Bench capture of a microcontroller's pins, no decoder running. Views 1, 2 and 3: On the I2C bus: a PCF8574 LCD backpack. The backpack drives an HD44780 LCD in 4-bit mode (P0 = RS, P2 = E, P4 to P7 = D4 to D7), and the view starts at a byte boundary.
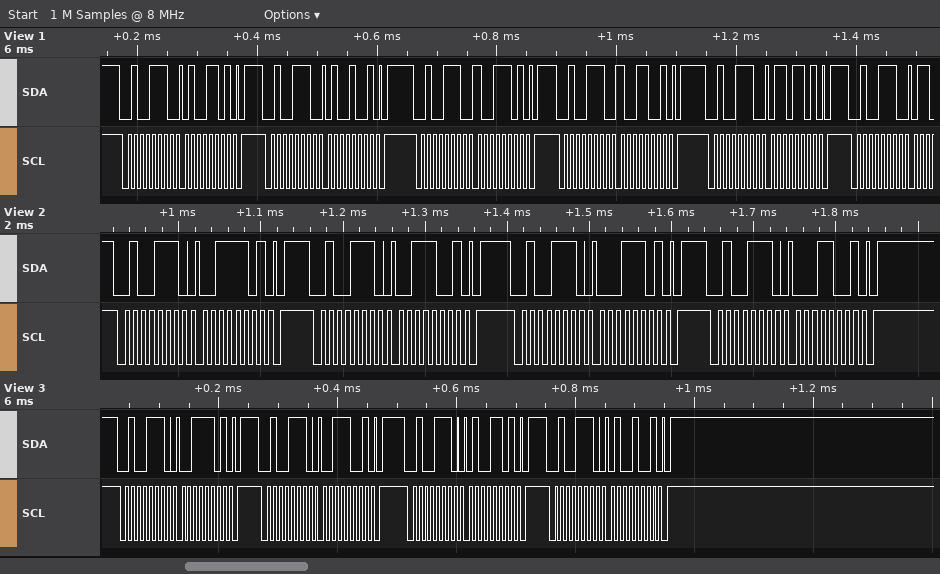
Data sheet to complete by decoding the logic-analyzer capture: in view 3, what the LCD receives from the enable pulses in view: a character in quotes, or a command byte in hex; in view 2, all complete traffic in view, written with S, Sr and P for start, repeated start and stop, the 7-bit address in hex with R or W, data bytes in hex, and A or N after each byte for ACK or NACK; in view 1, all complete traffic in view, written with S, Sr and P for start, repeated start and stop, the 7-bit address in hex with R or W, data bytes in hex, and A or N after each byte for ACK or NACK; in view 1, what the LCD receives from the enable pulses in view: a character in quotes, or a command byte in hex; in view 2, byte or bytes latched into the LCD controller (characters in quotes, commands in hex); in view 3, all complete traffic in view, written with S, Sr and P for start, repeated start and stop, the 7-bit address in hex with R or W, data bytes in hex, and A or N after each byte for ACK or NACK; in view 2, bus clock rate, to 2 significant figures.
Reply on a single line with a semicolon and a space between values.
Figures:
'4'; S 27W A 3D A P S 27W A 39 A P S 27W A 1D A P S 27W A 19 A P; S 27W A 4D A P S 27W A 49 A P S 27W A 9D A P S 27W A 99 A P S 27W A 6D A P S 27W A; 'I'; '1'; S 27W A 3D A P S 27W A 39 A P S 27W A 4D A P S 27W A 49 A P; 100 kHz
